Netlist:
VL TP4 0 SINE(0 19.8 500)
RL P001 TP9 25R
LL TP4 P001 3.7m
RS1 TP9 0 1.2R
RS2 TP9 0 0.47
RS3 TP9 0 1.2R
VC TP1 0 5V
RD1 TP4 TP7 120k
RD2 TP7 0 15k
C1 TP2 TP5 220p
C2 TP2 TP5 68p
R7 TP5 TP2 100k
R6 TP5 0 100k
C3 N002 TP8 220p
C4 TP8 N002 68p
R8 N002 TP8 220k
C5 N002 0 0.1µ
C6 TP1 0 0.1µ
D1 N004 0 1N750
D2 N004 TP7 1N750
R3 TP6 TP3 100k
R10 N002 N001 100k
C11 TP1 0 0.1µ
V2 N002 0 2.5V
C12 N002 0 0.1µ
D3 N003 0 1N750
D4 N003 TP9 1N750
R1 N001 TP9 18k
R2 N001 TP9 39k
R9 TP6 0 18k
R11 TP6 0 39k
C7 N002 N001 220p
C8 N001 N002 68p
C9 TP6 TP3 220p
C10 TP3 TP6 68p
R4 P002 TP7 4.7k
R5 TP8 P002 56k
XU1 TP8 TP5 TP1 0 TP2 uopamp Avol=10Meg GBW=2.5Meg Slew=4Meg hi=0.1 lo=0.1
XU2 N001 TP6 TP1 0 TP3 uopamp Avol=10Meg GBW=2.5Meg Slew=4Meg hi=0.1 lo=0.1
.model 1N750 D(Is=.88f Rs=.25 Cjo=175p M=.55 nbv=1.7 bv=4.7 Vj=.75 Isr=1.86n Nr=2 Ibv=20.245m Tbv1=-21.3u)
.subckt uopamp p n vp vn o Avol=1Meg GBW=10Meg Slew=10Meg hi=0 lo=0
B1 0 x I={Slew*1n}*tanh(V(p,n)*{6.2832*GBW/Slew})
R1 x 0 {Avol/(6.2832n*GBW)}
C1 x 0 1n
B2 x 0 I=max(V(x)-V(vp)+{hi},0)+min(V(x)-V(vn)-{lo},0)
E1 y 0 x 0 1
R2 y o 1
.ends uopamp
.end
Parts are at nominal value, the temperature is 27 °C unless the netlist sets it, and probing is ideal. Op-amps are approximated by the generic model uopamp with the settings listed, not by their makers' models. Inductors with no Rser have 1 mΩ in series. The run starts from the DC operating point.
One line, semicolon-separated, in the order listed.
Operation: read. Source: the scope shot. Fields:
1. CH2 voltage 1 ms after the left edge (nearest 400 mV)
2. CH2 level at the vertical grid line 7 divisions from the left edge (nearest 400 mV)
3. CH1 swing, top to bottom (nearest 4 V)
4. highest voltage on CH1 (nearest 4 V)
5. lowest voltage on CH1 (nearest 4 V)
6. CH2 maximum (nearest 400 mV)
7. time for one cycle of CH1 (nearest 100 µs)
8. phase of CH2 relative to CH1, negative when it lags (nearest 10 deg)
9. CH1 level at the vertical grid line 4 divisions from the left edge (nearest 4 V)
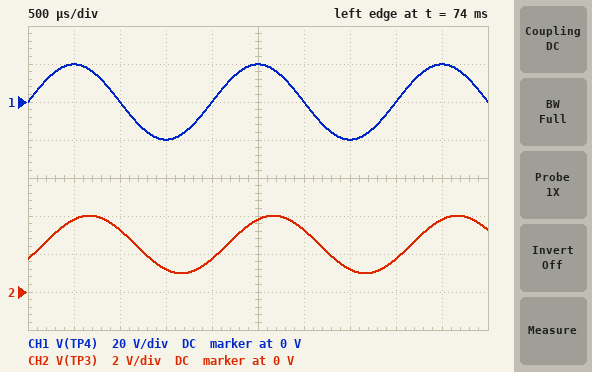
3.2 V; 1.2 V; 40 V; 20 V; -20 V; 4.0 V; 2.0 ms; -30 deg; 0 V
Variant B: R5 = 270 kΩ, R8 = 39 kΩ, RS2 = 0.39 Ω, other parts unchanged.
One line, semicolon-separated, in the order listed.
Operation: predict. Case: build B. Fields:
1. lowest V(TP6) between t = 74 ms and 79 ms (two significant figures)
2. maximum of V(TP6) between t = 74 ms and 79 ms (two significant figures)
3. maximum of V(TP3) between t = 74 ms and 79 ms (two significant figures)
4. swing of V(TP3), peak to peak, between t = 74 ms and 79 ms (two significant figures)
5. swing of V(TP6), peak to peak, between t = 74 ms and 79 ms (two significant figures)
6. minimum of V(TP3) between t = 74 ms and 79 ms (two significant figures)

120 mV; 420 mV; 3.9 V; 2.7 V; 300 mV; 1.1 V
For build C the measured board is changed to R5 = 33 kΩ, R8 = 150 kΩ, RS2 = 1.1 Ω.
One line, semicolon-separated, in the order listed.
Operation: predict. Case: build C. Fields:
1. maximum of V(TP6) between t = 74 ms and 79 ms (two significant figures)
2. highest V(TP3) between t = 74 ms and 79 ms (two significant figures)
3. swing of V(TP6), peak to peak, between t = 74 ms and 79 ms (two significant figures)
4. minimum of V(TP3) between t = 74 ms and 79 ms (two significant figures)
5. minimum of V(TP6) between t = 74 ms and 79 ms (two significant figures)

520 mV; 4.7 V; 490 mV; 270 mV; 29 mV
